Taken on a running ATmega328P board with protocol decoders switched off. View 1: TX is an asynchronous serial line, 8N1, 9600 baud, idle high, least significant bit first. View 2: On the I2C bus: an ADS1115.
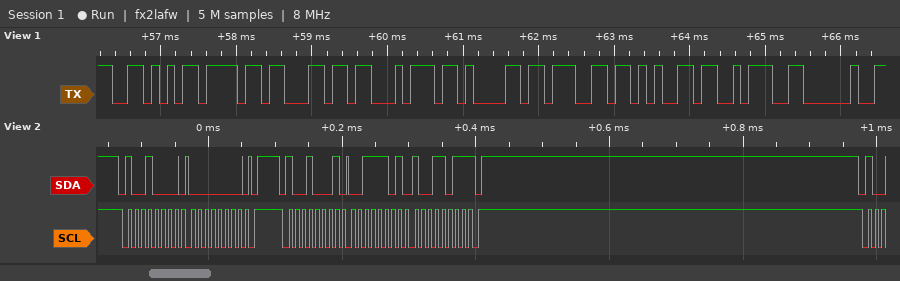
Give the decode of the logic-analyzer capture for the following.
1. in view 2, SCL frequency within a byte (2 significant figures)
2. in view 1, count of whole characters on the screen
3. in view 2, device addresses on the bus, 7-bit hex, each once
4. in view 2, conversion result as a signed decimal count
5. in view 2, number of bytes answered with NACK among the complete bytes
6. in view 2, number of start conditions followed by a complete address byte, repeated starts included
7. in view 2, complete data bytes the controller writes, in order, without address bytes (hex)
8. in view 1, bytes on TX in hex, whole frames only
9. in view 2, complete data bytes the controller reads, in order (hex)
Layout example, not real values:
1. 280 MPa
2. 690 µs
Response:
1. 100 kHz
2. 9
3. 0x48
4. 15771
5. 1
6. 2
7. 00
8. 56 6F 6C 74 61 67 65 3A 20
9. 3D 9B
